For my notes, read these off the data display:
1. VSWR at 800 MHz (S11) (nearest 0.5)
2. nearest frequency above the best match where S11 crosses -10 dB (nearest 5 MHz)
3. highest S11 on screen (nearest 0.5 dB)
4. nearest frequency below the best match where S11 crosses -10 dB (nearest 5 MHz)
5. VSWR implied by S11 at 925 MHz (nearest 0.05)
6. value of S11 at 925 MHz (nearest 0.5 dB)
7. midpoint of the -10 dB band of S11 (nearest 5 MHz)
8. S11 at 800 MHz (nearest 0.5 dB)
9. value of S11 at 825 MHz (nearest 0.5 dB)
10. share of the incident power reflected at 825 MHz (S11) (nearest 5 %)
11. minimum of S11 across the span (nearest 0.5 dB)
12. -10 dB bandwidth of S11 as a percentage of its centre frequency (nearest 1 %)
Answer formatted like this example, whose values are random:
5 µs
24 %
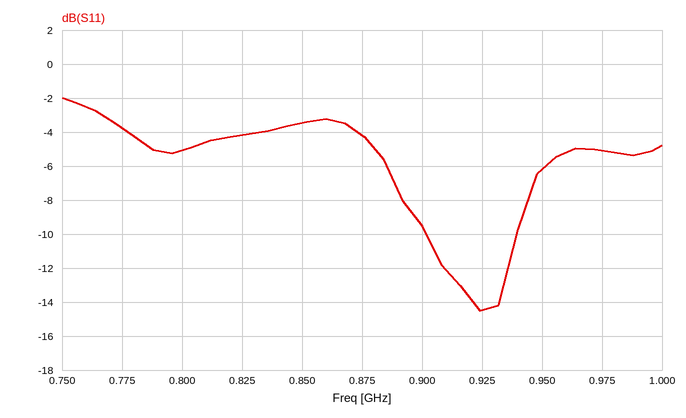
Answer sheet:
3.5
940 MHz
-2.0 dB
900 MHz
1.45
-14.5 dB
920 MHz
-5.0 dB
-4.0 dB
40 %
-14.5 dB
4 %
